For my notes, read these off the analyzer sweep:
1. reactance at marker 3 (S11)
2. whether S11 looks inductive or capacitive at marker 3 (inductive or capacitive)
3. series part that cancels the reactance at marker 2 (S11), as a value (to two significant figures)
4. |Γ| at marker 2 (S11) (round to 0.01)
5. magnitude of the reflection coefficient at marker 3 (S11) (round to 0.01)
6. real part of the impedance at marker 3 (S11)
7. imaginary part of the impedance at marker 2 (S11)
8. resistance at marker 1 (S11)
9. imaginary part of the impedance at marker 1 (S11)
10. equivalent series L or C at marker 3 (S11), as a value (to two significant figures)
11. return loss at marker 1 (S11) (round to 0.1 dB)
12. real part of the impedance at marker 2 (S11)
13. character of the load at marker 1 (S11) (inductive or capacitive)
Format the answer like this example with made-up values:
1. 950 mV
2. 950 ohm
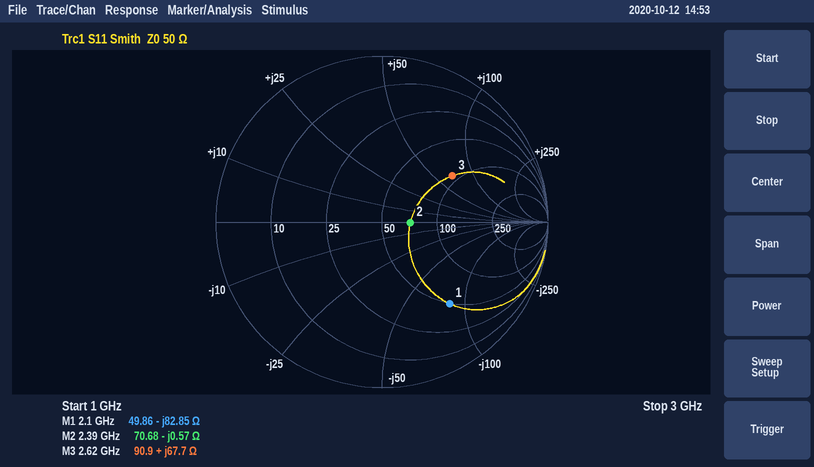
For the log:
1. +67.7 Ω
2. inductive
3. 38 pH
4. 0.17
5. 0.51
6. 90.9 Ω
7. -0.57 Ω
8. 49.86 Ω
9. -82.85 Ω
10. 4.1 nH
11. 3.9 dB
12. 70.68 Ω
13. capacitive
